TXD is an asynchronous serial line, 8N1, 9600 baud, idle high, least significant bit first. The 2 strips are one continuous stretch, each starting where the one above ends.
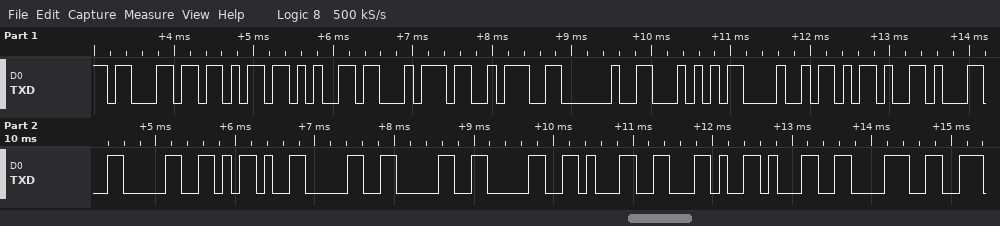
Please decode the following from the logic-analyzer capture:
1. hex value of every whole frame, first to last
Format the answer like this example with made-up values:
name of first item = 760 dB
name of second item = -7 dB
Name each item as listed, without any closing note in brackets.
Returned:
hex value of every whole frame, first to last = 63 6B 65 74 3A 20 54 48 2D 31 30 2D 30 30 30 31 2C 31 38
